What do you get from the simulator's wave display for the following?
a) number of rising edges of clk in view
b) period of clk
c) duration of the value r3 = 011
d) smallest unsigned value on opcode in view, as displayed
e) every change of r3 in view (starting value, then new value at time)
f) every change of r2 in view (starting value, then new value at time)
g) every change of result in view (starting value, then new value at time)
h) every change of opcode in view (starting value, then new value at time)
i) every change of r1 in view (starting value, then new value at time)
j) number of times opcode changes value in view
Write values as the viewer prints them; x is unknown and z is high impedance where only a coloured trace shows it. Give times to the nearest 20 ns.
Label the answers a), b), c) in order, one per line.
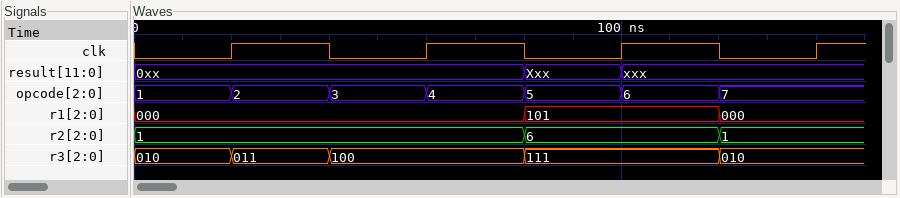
a) 4
b) 40 ns
c) 20 ns
d) 1
e) 010, 011 at 20 ns, 100 at 40 ns, 111 at 80 ns, 010 at 120 ns
f) 1, 6 at 80 ns, 1 at 120 ns
g) 0xx, Xxx at 80 ns, xxx at 100 ns
h) 1, 2 at 20 ns, 3 at 40 ns, 4 at 60 ns, 5 at 80 ns, 6 at 100 ns, 7 at 120 ns
i) 000, 101 at 80 ns, 000 at 120 ns
j) 6
